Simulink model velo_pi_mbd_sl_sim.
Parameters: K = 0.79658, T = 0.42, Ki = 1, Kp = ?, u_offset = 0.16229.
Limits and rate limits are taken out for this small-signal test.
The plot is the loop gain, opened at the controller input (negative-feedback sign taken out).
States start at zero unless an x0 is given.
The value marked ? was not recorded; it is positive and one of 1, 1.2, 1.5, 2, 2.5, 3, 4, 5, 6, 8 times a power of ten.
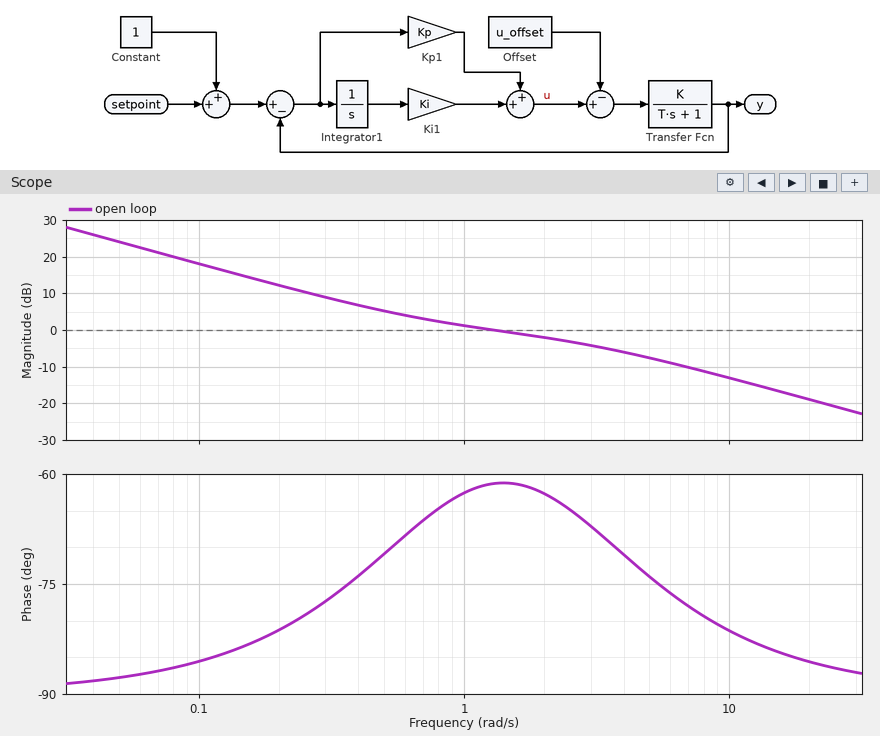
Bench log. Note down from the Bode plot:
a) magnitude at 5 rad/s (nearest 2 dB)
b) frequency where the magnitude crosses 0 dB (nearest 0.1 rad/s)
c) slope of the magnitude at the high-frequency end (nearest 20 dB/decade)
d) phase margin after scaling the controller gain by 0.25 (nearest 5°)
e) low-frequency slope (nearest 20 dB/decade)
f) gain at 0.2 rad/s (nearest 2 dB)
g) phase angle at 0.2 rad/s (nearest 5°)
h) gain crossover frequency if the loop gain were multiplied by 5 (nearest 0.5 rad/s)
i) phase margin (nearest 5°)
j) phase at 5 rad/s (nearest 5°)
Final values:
-8 dB
1.3 rad/s
-20 dB/decade
100°
-20 dB/decade
12 dB
-80°
11.0 rad/s
120°
-75°
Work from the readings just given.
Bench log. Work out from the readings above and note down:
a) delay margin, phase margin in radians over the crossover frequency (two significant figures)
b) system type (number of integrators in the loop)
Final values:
1.6 s
1
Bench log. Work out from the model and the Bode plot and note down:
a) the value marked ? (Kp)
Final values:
1.2
